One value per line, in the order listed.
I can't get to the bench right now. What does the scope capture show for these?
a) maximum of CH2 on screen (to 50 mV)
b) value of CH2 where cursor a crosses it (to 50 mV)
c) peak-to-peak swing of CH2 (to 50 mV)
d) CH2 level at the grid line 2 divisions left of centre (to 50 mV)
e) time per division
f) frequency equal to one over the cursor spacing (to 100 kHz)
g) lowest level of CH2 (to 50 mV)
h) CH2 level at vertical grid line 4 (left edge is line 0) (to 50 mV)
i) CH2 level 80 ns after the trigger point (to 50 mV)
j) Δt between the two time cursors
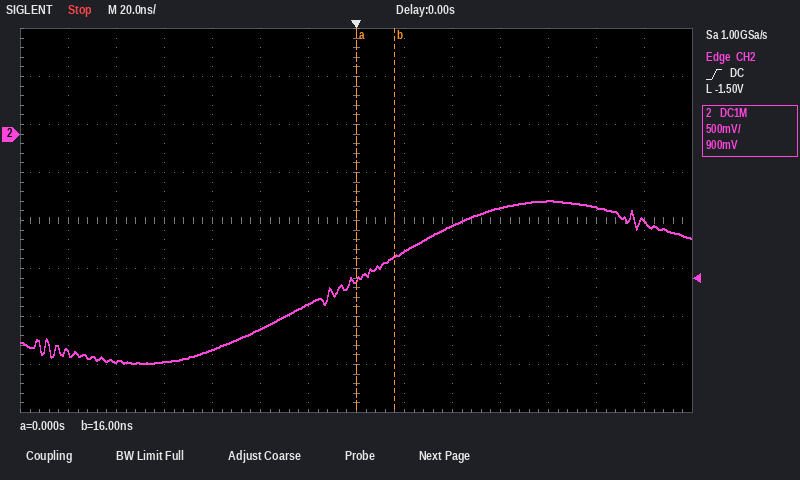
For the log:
-700 mV
-1.50 V
1.70 V
-2.05 V
20 ns
62.5 MHz
-2.40 V
-2.25 V
-700 mV
16 ns
